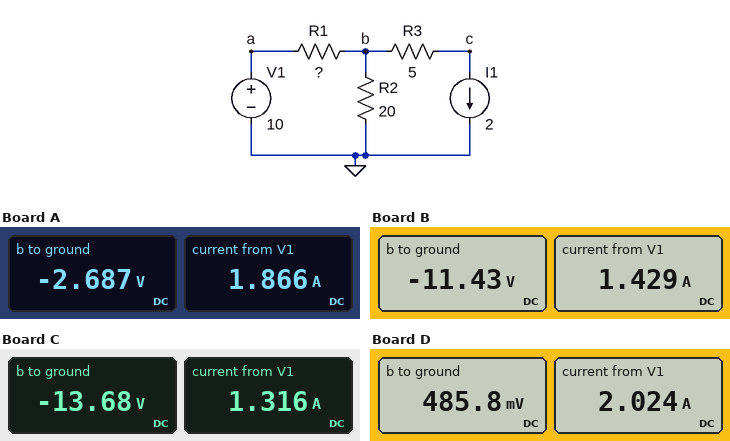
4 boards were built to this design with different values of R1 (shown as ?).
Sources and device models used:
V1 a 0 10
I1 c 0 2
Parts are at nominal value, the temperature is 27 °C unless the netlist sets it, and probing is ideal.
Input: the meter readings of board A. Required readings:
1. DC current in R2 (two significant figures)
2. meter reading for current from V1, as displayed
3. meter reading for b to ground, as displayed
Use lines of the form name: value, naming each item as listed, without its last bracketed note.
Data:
DC current in R2: 130 mA
meter reading for current from V1, as displayed: 1.866 A
meter reading for b to ground, as displayed: -2.687 V
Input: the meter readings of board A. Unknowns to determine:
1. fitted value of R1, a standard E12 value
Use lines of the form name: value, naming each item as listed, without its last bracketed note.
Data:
fitted value of R1, a standard E12 value: 6.8 Ω
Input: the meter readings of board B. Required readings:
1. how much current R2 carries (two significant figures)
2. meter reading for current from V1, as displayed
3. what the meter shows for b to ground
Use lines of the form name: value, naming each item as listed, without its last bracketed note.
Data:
how much current R2 carries: 570 mA
meter reading for current from V1, as displayed: 1.429 A
what the meter shows for b to ground: -11.43 V
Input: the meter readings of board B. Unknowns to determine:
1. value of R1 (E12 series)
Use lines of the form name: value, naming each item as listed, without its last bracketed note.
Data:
value of R1: 15 Ω
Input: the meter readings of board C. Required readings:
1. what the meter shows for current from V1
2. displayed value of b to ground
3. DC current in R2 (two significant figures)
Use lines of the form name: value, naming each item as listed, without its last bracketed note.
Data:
what the meter shows for current from V1: 1.316 A
displayed value of b to ground: -13.68 V
DC current in R2: 680 mA
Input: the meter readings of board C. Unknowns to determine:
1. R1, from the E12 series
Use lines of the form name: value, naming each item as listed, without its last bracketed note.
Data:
R1, from the E12 series: 18 Ω
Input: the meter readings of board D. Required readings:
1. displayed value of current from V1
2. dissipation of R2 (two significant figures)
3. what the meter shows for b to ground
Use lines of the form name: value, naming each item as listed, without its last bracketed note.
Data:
displayed value of current from V1: 2.024 A
dissipation of R2: 12 mW
what the meter shows for b to ground: 485.8 mV
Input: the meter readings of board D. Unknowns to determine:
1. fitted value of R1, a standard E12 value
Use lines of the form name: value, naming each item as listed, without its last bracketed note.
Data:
fitted value of R1, a standard E12 value: 4.7 Ω
